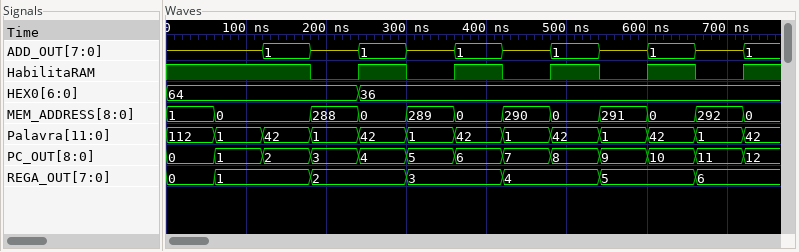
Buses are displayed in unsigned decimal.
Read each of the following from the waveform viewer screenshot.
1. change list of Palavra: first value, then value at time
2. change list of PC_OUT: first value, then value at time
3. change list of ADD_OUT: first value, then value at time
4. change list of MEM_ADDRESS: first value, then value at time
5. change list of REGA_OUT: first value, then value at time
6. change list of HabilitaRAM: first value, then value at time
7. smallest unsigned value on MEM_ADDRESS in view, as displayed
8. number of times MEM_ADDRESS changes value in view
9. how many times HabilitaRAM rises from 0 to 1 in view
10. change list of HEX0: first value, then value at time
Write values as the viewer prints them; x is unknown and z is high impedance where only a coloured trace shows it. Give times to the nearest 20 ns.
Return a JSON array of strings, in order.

["112, 1 at 60 ns, 42 at 120 ns, 1 at 180 ns, 42 at 240 ns, 1 at 300 ns, 42 at 360 ns, 1 at 420 ns, 42 at 480 ns, 1 at 540 ns, 42 at 600 ns, 1 at 660 ns, 42 at 720 ns", "0, 1 at 60 ns, 2 at 120 ns, 3 at 180 ns, 4 at 240 ns, 5 at 300 ns, 6 at 360 ns, 7 at 420 ns, 8 at 480 ns, 9 at 540 ns, 10 at 600 ns, 11 at 660 ns, 12 at 720 ns", "z, 1 at 120 ns, z at 180 ns, 1 at 240 ns, z at 300 ns, 1 at 360 ns, z at 420 ns, 1 at 480 ns, z at 540 ns, 1 at 600 ns, z at 660 ns, 1 at 720 ns", "1, 0 at 60 ns, 288 at 180 ns, 0 at 240 ns, 289 at 300 ns, 0 at 360 ns, 290 at 420 ns, 0 at 480 ns, 291 at 540 ns, 0 at 600 ns, 292 at 660 ns, 0 at 720 ns", "0, 1 at 60 ns, 2 at 180 ns, 3 at 300 ns, 4 at 420 ns, 5 at 540 ns, 6 at 660 ns", "1, 0 at 180 ns, 1 at 240 ns, 0 at 300 ns, 1 at 360 ns, 0 at 420 ns, 1 at 480 ns, 0 at 540 ns, 1 at 600 ns, 0 at 660 ns, 1 at 720 ns", "0", "11", "5", "64, 36 at 240 ns"]
